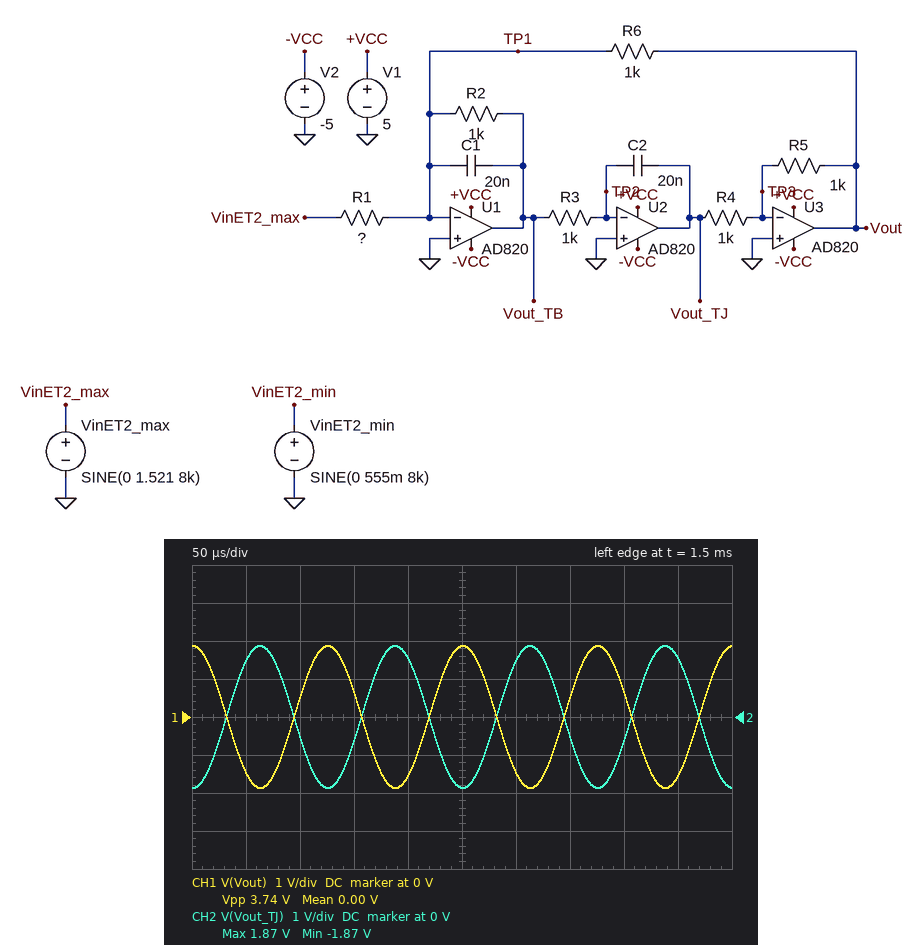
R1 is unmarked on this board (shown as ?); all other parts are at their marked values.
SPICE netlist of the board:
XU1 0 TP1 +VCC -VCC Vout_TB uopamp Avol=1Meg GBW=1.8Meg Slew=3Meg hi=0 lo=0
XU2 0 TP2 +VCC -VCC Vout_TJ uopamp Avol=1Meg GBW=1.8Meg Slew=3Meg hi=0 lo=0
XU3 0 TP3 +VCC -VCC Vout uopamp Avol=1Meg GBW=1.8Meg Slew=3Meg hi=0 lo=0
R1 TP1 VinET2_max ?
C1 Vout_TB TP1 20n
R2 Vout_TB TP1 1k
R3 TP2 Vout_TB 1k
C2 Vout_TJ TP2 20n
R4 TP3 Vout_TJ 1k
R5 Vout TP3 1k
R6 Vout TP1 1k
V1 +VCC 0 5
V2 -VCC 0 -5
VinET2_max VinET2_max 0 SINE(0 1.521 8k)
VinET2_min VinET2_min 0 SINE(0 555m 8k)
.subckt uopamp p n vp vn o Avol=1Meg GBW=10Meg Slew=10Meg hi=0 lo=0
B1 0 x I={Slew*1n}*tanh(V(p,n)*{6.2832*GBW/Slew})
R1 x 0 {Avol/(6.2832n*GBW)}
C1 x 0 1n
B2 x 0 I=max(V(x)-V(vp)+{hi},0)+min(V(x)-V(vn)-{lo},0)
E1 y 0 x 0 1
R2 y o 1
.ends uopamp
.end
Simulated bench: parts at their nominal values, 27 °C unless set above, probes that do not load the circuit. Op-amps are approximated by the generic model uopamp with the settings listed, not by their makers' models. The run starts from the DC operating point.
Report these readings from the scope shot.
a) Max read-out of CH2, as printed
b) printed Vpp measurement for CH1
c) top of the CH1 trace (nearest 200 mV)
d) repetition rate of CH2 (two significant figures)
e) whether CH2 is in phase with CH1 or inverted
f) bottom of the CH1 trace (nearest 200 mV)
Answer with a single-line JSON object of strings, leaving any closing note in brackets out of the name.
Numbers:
{"Max read-out of CH2, as printed": "1.87 V", "printed Vpp measurement for CH1": "3.74 V", "top of the CH1 trace": "1.8 V", "repetition rate of CH2": "8.0 kHz", "whether CH2 is in phase with CH1 or inverted": "inverted", "bottom of the CH1 trace": "-1.8 V"}
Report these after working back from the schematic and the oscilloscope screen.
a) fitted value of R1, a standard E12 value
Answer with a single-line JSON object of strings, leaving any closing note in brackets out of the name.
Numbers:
{"fitted value of R1, a standard E12 value": "820 Ω"}
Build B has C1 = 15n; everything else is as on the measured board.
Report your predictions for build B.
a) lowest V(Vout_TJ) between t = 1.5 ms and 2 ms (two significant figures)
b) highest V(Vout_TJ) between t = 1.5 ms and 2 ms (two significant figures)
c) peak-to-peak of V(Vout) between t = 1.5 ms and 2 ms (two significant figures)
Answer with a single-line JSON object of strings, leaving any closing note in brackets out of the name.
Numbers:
{"lowest V(Vout_TJ) between t = 1.5 ms and 2 ms": "-1.8 V", "highest V(Vout_TJ) between t = 1.5 ms and 2 ms": "1.8 V", "peak-to-peak of V(Vout) between t = 1.5 ms and 2 ms": "3.6 V"}
